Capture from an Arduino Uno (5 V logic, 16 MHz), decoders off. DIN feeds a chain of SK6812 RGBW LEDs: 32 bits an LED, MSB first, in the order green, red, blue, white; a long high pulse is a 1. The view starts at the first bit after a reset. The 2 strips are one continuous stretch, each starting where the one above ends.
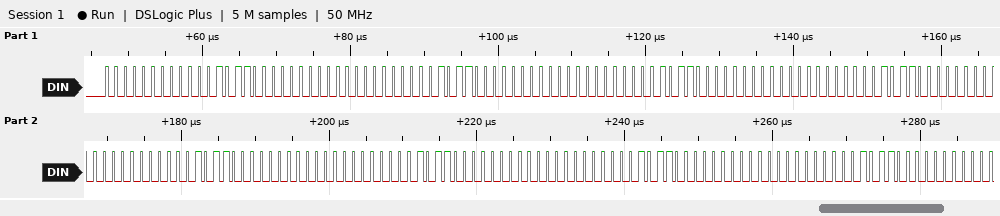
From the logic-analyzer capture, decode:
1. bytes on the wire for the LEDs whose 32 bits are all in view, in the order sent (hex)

00 0B 00 00 0B 00 00 0B 00 00 0B 00 00 0B 00 00 0B 00 00 0B 00 00 0B 00
